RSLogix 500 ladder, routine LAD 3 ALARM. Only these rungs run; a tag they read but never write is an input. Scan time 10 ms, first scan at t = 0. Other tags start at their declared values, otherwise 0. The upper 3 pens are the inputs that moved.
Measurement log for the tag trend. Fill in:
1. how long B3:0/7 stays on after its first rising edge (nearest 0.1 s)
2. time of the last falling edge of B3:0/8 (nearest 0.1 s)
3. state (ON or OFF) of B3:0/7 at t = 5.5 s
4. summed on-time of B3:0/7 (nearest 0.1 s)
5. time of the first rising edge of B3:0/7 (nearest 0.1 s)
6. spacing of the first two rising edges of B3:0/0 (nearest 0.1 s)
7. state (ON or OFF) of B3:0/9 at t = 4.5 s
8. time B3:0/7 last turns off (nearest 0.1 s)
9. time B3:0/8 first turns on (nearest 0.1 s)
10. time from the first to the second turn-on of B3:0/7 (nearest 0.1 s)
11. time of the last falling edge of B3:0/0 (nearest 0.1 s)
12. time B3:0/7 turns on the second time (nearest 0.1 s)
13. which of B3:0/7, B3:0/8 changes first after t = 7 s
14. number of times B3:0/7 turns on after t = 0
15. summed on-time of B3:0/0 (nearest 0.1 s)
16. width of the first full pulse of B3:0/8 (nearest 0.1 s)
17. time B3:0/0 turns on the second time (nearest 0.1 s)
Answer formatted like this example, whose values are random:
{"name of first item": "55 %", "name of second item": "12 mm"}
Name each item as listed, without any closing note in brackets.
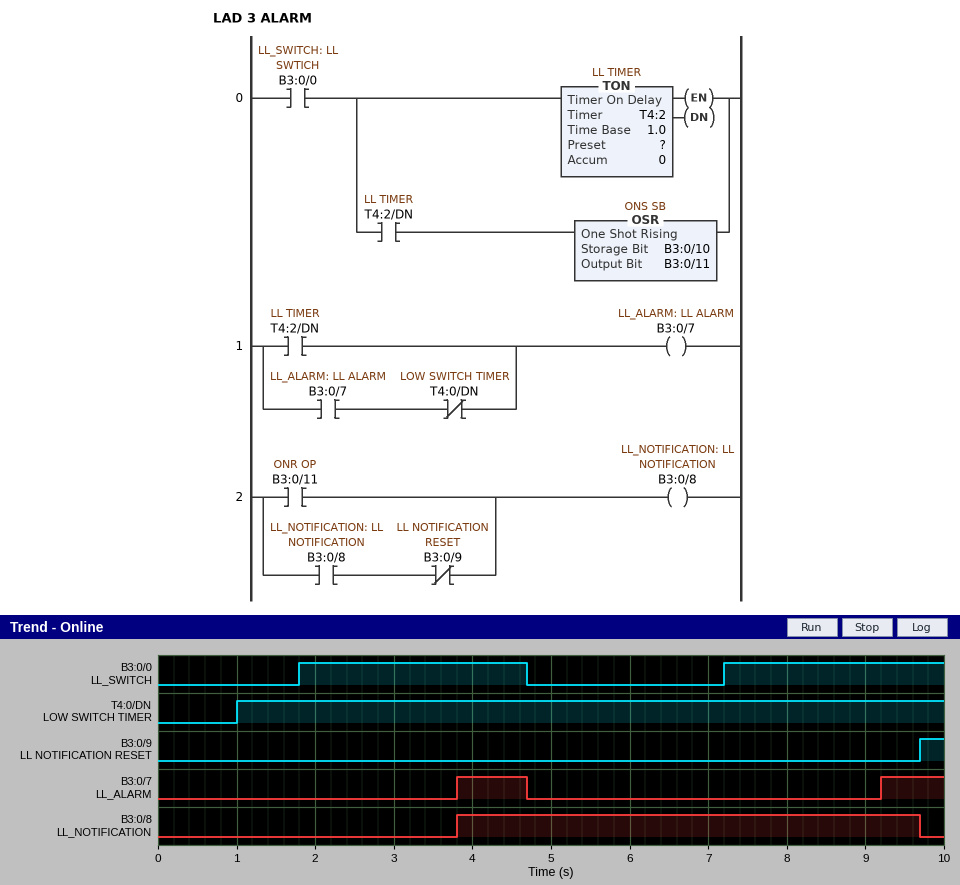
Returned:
{"how long B3:0/7 stays on after its first rising edge": "0.9 s", "time of the last falling edge of B3:0/8": "9.7 s", "state (ON or OFF) of B3:0/7 at t = 5.5 s": "OFF", "summed on-time of B3:0/7": "1.7 s", "time of the first rising edge of B3:0/7": "3.8 s", "spacing of the first two rising edges of B3:0/0": "5.4 s", "state (ON or OFF) of B3:0/9 at t = 4.5 s": "OFF", "time B3:0/7 last turns off": "4.7 s", "time B3:0/8 first turns on": "3.8 s", "time from the first to the second turn-on of B3:0/7": "5.4 s", "time of the last falling edge of B3:0/0": "4.7 s", "time B3:0/7 turns on the second time": "9.2 s", "which of B3:0/7, B3:0/8 changes first after t = 7 s": "B3:0/7", "number of times B3:0/7 turns on after t = 0": "2", "summed on-time of B3:0/0": "5.7 s", "width of the first full pulse of B3:0/8": "5.9 s", "time B3:0/0 turns on the second time": "7.2 s"}
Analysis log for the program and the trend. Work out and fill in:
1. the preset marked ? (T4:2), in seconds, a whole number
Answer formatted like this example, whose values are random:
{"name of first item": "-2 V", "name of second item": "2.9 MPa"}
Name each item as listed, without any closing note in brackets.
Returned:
{"the preset marked ? (T4:2), in seconds, a whole number": "2 s"}
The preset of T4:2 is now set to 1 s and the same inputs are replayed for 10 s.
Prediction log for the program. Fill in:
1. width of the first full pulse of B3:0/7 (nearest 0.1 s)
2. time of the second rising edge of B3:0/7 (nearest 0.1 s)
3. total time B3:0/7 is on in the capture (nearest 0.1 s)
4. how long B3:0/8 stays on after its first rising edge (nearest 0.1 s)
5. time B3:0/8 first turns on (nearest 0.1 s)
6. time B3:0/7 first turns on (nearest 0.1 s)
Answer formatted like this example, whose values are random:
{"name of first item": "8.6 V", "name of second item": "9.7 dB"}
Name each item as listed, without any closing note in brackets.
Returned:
{"width of the first full pulse of B3:0/7": "1.9 s", "time of the second rising edge of B3:0/7": "8.2 s", "total time B3:0/7 is on in the capture": "3.7 s", "how long B3:0/8 stays on after its first rising edge": "6.9 s", "time B3:0/8 first turns on": "2.8 s", "time B3:0/7 first turns on": "2.8 s"}
